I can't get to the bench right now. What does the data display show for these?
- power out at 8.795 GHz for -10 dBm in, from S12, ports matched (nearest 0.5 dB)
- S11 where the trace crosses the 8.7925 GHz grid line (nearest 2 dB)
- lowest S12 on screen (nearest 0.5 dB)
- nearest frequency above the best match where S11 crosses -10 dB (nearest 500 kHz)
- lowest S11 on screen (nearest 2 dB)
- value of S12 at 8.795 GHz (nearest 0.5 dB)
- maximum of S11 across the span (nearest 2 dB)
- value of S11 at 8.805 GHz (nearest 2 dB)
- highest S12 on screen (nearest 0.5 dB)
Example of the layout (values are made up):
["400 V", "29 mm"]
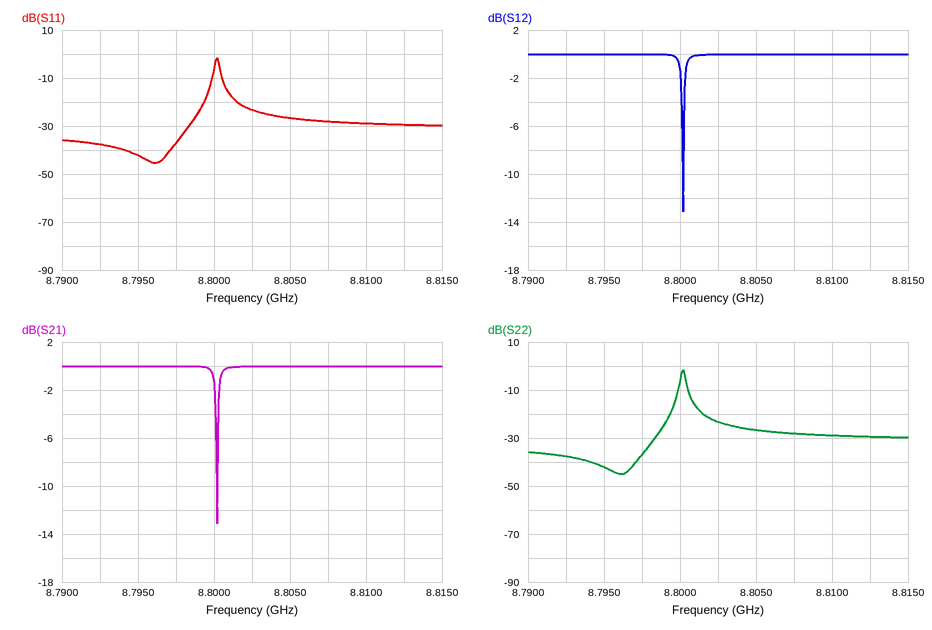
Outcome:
["-10.0 dBm", "-38 dB", "-13.0 dB", "8.8000 GHz", "-46 dB", "0.0 dB", "-2 dB", "-26 dB", "0.0 dB"]
